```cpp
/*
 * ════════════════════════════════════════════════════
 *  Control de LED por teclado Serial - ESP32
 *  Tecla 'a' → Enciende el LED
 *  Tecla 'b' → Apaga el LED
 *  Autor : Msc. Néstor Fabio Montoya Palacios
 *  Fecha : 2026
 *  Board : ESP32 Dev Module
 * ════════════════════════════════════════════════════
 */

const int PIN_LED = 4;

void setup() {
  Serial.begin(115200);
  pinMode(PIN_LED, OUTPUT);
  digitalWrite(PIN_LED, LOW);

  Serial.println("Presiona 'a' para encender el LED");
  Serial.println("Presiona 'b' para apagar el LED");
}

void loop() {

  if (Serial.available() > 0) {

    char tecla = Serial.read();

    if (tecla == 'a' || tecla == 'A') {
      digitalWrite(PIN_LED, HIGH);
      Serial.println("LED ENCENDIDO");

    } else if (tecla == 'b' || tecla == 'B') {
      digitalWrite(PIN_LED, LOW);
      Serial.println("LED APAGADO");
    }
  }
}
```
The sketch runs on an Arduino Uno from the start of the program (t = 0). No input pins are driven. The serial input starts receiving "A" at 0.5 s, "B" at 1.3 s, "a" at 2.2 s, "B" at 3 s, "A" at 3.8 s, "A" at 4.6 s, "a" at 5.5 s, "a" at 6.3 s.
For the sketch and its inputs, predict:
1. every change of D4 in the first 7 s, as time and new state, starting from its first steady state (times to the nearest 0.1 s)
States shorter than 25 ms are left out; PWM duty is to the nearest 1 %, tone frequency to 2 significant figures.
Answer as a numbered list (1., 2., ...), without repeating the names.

1. 0 s low; 0.5 s high; 1.3 s low; 2.2 s high; 3 s low; 3.8 s high
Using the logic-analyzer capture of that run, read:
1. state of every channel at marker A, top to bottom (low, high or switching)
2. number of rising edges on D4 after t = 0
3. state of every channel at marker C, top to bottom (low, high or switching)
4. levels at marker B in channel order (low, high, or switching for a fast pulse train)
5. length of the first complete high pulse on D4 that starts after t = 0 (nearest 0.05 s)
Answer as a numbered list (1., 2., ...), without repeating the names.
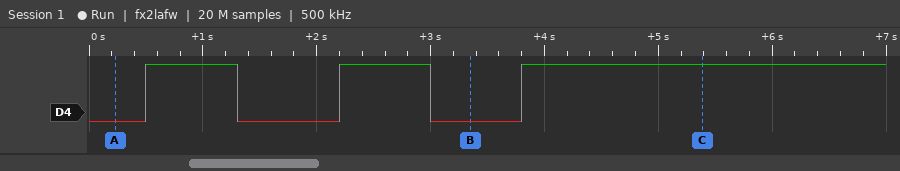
1. D4 low
2. 3
3. D4 high
4. D4 low
5. 0.80 s
